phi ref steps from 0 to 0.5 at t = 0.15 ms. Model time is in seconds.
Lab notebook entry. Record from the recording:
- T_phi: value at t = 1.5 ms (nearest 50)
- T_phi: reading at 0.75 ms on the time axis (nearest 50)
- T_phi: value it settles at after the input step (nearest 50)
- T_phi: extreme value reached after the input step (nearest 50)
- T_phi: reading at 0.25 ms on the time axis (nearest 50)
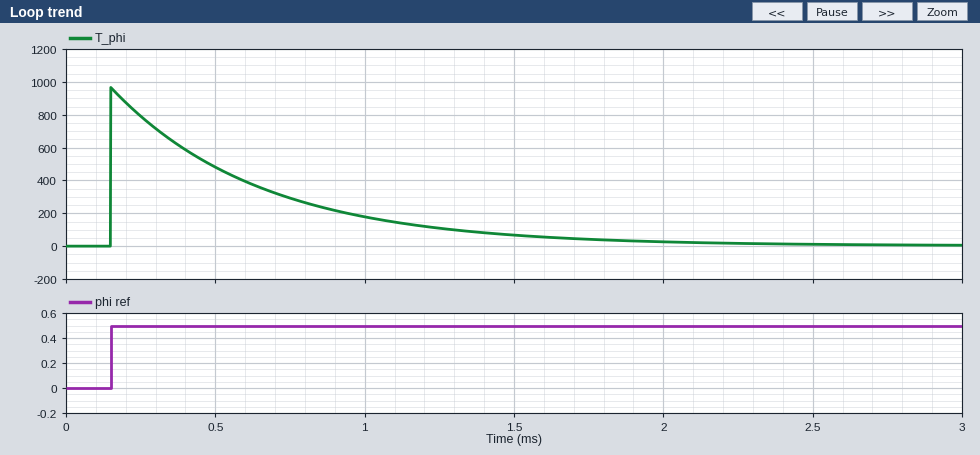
50
300
0
950
800
